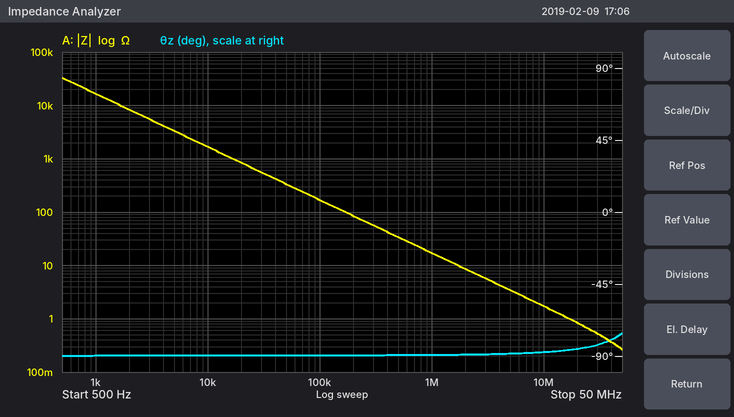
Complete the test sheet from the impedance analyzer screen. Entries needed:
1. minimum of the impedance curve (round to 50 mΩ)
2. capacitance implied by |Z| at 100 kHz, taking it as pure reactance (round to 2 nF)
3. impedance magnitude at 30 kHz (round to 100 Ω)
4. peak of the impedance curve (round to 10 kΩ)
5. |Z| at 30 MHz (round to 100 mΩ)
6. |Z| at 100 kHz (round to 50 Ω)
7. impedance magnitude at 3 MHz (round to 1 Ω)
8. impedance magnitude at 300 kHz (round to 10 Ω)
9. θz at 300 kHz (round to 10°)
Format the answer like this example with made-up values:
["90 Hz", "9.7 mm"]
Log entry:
["250 mΩ", "10 nF", "600 Ω", "30 kΩ", "500 mΩ", "150 Ω", "6 Ω", "60 Ω", "-90°"]
